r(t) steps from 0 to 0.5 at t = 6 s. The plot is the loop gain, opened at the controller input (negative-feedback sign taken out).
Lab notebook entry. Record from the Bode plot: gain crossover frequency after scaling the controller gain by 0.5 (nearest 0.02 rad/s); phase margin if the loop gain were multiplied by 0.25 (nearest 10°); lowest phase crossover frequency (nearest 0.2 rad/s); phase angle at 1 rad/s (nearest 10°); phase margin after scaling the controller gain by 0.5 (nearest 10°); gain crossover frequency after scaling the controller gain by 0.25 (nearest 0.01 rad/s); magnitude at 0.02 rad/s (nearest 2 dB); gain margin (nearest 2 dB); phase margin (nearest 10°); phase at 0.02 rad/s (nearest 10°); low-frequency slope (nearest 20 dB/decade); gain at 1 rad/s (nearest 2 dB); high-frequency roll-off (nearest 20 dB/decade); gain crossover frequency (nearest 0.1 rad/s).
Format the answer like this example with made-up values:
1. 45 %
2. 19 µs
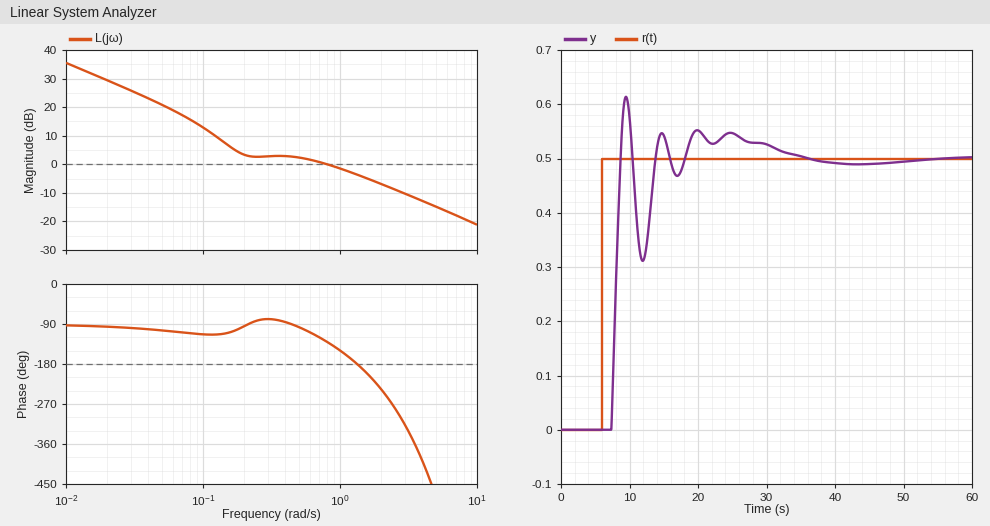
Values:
1. 0.16 rad/s
2. 70°
3. 1.4 rad/s
4. -150°
5. 70°
6. 0.11 rad/s
7. 30 dB
8. 4 dB
9. 50°
10. -100°
11. -20 dB/decade
12. -2 dB
13. -20 dB/decade
14. 0.8 rad/s
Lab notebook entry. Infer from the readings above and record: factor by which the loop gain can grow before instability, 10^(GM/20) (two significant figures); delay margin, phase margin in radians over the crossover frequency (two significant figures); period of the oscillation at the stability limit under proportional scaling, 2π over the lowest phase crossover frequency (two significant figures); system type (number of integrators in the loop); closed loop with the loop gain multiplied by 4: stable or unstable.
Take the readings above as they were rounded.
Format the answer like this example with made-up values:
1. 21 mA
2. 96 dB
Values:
1. 1.6
2. 1.1 s
3. 4.5 s
4. 1
5. unstable
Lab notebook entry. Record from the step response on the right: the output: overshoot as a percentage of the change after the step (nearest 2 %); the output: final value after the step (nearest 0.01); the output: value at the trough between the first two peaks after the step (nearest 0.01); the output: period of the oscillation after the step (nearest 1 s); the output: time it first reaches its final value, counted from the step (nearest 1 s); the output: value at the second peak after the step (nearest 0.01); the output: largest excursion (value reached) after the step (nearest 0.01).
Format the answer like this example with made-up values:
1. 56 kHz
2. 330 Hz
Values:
1. 22 %
2. 0.50
3. 0.31
4. 5 s
5. 3 s
6. 0.55
7. 0.61
